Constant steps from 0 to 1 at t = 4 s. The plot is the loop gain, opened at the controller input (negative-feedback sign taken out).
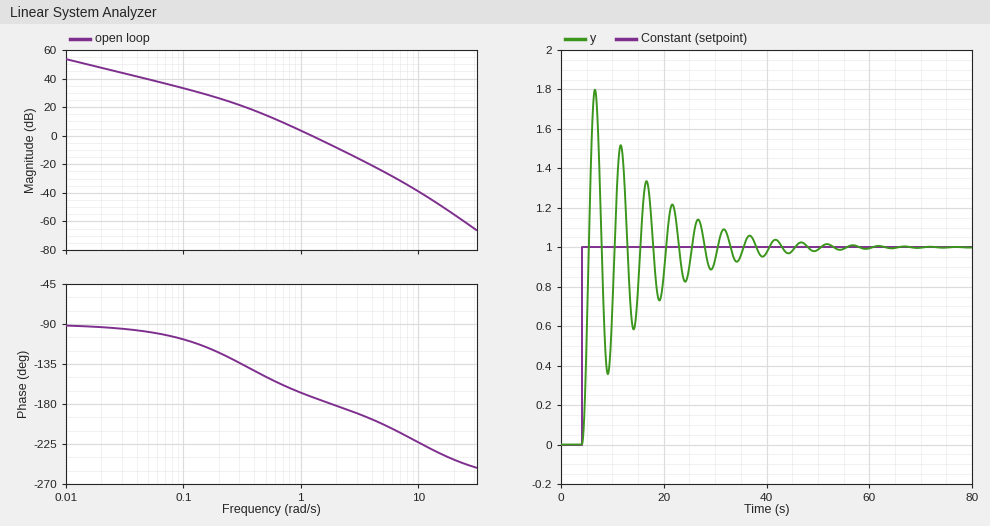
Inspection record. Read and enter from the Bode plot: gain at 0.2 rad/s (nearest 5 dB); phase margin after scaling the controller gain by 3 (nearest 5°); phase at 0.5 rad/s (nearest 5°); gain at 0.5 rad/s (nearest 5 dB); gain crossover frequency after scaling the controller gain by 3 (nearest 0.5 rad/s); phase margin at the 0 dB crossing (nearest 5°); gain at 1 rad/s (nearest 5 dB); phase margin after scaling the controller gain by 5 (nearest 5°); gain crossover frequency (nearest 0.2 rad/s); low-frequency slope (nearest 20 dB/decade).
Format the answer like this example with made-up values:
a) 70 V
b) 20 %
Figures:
a) 25 dB
b) -5°
c) -150°
d) 15 dB
e) 2.0 rad/s
f) 10°
g) 5 dB
h) -10°
i) 1.2 rad/s
j) -20 dB/decade
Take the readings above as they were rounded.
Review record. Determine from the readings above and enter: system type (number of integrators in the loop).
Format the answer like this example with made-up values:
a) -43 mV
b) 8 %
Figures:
a) 1
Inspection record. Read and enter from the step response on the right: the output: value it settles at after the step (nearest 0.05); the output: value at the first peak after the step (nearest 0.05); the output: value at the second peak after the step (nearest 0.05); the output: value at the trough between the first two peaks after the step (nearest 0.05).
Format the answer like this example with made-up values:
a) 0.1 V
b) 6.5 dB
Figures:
a) 1.00
b) 1.80
c) 1.50
d) 0.35
